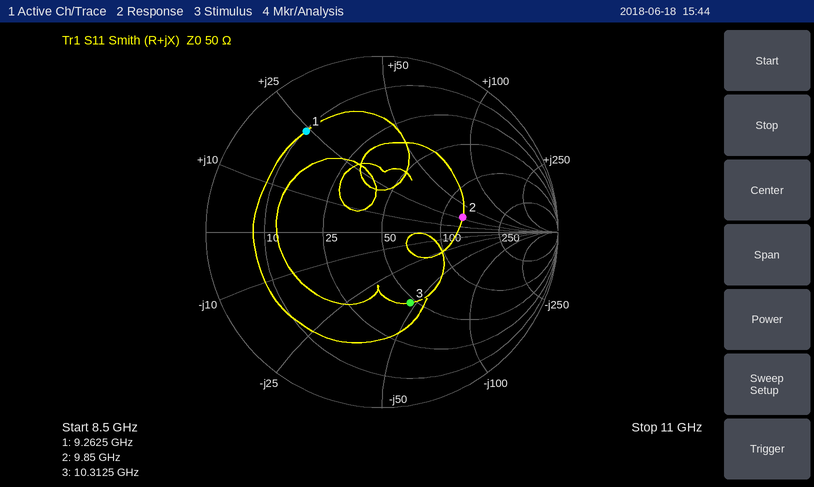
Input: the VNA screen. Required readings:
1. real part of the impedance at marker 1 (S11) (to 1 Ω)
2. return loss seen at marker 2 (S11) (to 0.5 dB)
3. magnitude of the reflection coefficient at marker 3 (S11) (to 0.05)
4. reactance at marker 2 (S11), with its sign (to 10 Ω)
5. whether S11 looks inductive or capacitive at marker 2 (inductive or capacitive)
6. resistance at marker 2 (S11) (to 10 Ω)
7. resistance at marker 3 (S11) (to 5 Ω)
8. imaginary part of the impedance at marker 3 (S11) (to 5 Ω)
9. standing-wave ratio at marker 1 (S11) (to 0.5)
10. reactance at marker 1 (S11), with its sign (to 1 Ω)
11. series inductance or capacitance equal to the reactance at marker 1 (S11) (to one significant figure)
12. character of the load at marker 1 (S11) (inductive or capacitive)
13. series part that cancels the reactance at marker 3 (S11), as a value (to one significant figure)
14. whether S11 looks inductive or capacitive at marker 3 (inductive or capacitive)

10 Ω
6.5 dB
0.45
+30 Ω
inductive
130 Ω
45 Ω
-45 Ω
6.0
+24 Ω
400 pH
inductive
700 pH
capacitive
